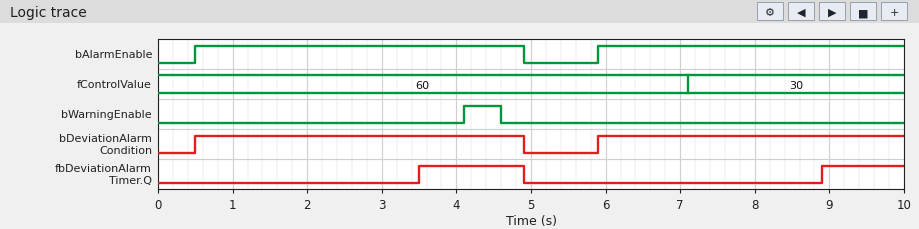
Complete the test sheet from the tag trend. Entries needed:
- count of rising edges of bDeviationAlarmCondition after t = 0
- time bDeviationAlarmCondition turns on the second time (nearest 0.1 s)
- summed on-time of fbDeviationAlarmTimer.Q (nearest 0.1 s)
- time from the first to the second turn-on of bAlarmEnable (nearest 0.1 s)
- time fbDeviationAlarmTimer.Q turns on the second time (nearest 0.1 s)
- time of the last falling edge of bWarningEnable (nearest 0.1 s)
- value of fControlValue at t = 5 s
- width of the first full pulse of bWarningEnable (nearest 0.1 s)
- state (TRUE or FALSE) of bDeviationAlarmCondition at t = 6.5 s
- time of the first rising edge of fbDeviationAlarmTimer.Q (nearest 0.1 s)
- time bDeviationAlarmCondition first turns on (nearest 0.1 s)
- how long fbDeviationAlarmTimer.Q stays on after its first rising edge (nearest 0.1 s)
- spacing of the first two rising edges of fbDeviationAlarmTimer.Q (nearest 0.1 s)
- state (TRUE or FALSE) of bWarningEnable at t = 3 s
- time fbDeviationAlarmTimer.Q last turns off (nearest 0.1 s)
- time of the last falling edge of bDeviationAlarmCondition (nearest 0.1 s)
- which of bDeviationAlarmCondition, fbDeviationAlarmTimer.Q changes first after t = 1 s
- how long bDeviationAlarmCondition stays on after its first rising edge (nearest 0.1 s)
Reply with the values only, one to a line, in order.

2
5.9 s
2.5 s
5.4 s
8.9 s
4.6 s
60
0.5 s
TRUE
3.5 s
0.5 s
1.4 s
5.4 s
FALSE
4.9 s
4.9 s
fbDeviationAlarmTimer.Q
4.4 s
